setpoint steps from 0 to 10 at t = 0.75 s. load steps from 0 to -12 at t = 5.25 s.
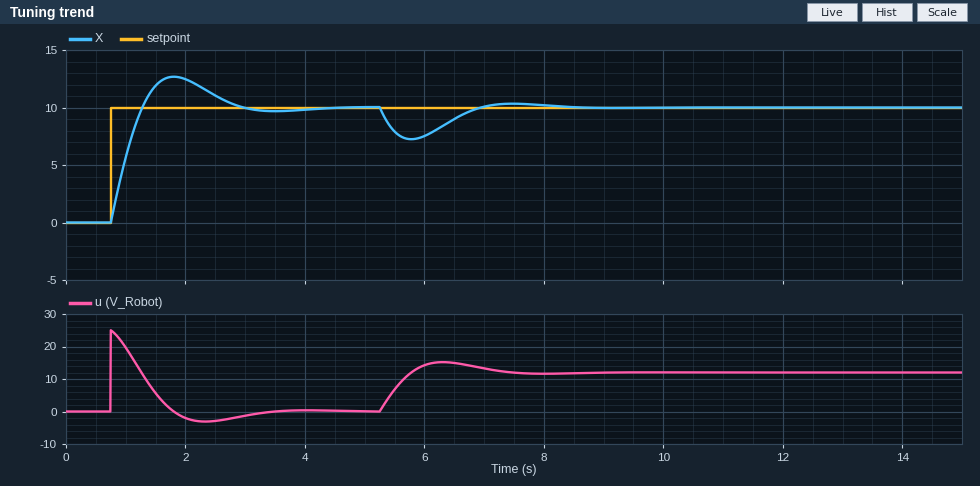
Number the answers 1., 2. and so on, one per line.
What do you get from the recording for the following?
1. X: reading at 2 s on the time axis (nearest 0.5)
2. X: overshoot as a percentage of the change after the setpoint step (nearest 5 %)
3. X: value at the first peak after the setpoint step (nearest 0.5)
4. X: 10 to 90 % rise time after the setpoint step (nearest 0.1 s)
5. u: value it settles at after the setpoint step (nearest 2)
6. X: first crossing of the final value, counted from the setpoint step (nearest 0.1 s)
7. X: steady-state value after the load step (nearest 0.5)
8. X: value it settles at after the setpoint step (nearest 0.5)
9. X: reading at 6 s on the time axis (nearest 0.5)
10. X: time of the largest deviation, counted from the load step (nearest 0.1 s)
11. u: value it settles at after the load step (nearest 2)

1. 12.5
2. 25 %
3. 12.5
4. 0.4 s
5. 0
6. 0.5 s
7. 10.0
8. 10.0
9. 7.5
10. 0.5 s
11. 12
